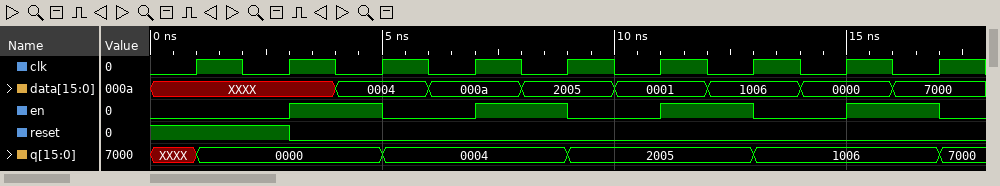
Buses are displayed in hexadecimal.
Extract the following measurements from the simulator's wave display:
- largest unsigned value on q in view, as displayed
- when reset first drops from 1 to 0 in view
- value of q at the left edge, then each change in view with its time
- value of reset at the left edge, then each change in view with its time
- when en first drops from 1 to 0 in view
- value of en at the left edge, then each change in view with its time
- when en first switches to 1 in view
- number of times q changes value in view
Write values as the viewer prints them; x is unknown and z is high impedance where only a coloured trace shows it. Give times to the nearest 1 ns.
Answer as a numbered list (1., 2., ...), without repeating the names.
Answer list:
1. 7000
2. 3 ns
3. XXXX, 0000 at 1 ns, 0004 at 5 ns, 2005 at 9 ns, 1006 at 13 ns, 7000 at 17 ns
4. 1, 0 at 3 ns
5. 5 ns
6. 0, 1 at 3 ns, 0 at 5 ns, 1 at 7 ns, 0 at 9 ns, 1 at 11 ns, 0 at 13 ns, 1 at 15 ns, 0 at 17 ns
7. 3 ns
8. 5
